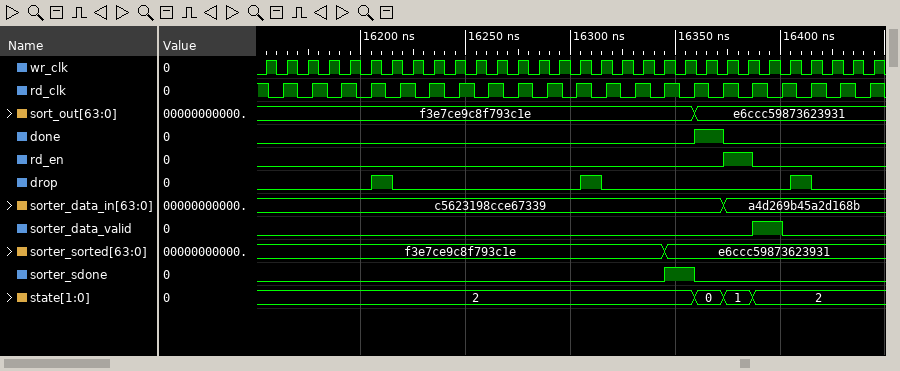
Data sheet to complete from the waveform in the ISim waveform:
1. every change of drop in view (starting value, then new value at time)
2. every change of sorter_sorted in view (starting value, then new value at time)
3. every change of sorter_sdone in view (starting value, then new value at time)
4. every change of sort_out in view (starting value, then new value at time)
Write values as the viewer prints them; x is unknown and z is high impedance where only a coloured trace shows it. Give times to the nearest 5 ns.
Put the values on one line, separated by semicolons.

0, 1 at 16205 ns, 0 at 16215 ns, 1 at 16305 ns, 0 at 16315 ns, 1 at 16405 ns, 0 at 16415 ns; f3e7ce9c8f793c1e, e6ccc59873623931 at 16345 ns; 0, 1 at 16345 ns, 0 at 16360 ns; f3e7ce9c8f793c1e, e6ccc59873623931 at 16360 ns
